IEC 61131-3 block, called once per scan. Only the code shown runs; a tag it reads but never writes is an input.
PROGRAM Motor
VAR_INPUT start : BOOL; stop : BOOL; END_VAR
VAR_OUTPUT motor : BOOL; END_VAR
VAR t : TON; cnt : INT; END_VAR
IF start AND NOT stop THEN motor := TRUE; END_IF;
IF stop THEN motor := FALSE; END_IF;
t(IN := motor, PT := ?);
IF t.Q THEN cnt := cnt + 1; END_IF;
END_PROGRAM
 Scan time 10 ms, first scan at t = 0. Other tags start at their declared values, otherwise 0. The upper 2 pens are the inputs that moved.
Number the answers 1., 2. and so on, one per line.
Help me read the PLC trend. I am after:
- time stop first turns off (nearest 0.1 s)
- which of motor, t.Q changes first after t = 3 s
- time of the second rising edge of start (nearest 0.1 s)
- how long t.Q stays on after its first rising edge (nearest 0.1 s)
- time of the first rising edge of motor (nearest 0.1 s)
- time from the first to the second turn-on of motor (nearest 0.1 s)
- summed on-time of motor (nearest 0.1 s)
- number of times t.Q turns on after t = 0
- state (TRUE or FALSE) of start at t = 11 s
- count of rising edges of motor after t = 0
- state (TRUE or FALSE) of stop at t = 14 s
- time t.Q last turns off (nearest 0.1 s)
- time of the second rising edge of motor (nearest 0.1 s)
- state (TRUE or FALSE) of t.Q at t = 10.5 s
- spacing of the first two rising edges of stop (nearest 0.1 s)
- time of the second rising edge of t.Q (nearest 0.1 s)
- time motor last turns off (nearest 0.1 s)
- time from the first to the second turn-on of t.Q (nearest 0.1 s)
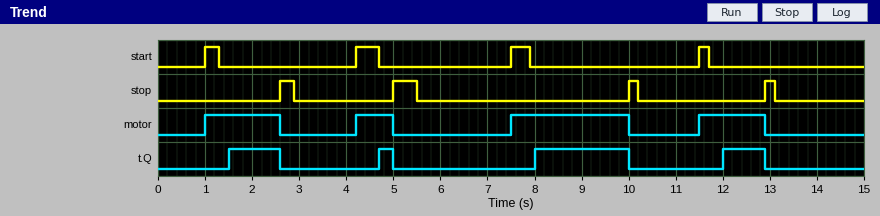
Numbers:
1. 2.9 s
2. motor
3. 4.2 s
4. 1.1 s
5. 1.0 s
6. 3.2 s
7. 6.3 s
8. 4
9. FALSE
10. 4
11. FALSE
12. 12.9 s
13. 4.2 s
14. FALSE
15. 2.4 s
16. 4.7 s
17. 12.9 s
18. 3.2 s
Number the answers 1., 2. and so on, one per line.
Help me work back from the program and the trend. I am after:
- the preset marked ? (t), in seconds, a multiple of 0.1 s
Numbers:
1. 0.5 s
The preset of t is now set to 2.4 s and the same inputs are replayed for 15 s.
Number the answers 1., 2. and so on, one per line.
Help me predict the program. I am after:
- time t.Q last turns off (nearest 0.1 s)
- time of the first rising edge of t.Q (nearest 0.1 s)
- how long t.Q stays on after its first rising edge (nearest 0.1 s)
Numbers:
1. 10.0 s
2. 9.9 s
3. 0.1 s
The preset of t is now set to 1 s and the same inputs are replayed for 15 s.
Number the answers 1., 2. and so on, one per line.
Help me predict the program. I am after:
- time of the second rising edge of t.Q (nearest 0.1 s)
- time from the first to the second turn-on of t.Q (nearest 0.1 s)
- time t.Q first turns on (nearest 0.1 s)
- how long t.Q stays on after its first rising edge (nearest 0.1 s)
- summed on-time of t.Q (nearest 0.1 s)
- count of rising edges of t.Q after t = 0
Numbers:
1. 8.5 s
2. 6.5 s
3. 2.0 s
4. 0.6 s
5. 2.5 s
6. 3
